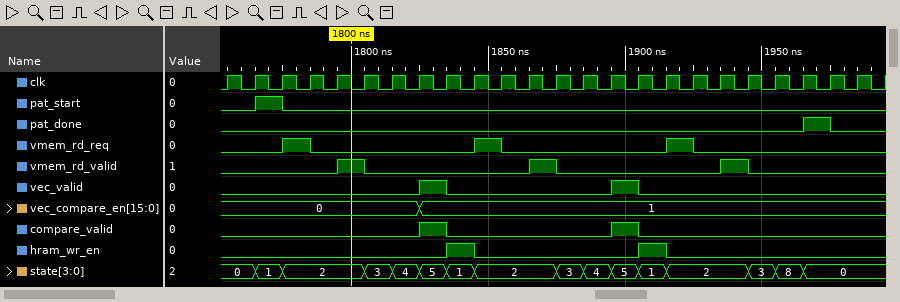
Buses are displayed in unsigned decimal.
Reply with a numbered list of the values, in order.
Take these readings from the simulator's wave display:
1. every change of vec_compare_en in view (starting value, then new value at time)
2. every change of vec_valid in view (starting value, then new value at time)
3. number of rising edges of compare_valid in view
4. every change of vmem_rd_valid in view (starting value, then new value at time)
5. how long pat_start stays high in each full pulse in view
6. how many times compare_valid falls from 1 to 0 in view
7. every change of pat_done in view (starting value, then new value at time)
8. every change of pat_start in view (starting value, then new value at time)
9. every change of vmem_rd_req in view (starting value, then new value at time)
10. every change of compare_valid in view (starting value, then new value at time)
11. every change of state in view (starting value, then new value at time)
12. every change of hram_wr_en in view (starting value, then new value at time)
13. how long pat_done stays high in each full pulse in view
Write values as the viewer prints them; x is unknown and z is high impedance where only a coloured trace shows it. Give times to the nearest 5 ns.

1. 0, 1 at 1825 ns
2. 0, 1 at 1825 ns, 0 at 1835 ns, 1 at 1895 ns, 0 at 1905 ns
3. 2
4. 0, 1 at 1795 ns, 0 at 1805 ns, 1 at 1865 ns, 0 at 1875 ns, 1 at 1935 ns, 0 at 1945 ns
5. 10 ns
6. 2
7. 0, 1 at 1965 ns, 0 at 1975 ns
8. 0, 1 at 1765 ns, 0 at 1775 ns
9. 0, 1 at 1775 ns, 0 at 1785 ns, 1 at 1845 ns, 0 at 1855 ns, 1 at 1915 ns, 0 at 1925 ns
10. 0, 1 at 1825 ns, 0 at 1835 ns, 1 at 1895 ns, 0 at 1905 ns
11. 0, 1 at 1765 ns, 2 at 1775 ns, 3 at 1805 ns, 4 at 1815 ns, 5 at 1825 ns, 1 at 1835 ns, 2 at 1845 ns, 3 at 1875 ns, 4 at 1885 ns, 5 at 1895 ns, 1 at 1905 ns, 2 at 1915 ns, 3 at 1945 ns, 8 at 1955 ns, 0 at 1965 ns
12. 0, 1 at 1835 ns, 0 at 1845 ns, 1 at 1905 ns, 0 at 1915 ns
13. 10 ns
